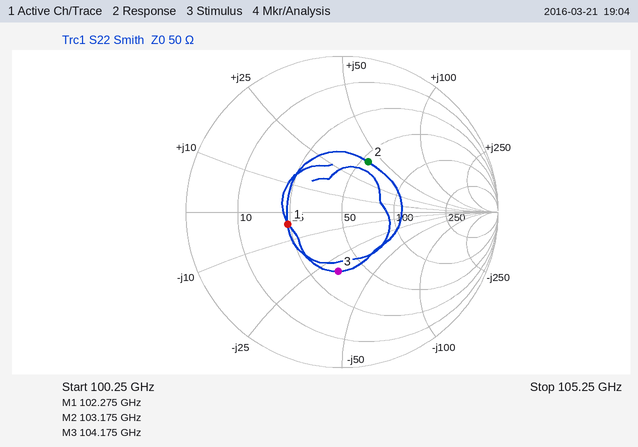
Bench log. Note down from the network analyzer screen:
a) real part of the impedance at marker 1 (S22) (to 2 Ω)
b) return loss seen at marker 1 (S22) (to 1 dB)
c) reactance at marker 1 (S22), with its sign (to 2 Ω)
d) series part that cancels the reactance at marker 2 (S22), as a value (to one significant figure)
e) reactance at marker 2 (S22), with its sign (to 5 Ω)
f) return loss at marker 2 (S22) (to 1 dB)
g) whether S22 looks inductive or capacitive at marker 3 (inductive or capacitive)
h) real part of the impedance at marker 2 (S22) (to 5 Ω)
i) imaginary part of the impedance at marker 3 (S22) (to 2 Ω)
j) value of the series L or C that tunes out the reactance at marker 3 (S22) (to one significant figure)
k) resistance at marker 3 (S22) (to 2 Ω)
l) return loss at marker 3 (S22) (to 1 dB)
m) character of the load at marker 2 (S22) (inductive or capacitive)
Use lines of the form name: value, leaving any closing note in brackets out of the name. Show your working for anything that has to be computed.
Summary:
real part of the impedance at marker 1 (S22): 24 Ω
return loss seen at marker 1 (S22): 9 dB
reactance at marker 1 (S22), with its sign: -4 Ω
series part that cancels the reactance at marker 2 (S22), as a value: C = 1/(2π × 103.175 GHz × 40 Ω) ≈ 38.6 fF, so 40 fF to one significant figure
reactance at marker 2 (S22), with its sign: +40 Ω
return loss at marker 2 (S22): 9 dB
whether S22 looks inductive or capacitive at marker 3: capacitive
real part of the impedance at marker 2 (S22): 55 Ω
imaginary part of the impedance at marker 3 (S22): -32 Ω
value of the series L or C that tunes out the reactance at marker 3 (S22): L = 32 Ω/(2π × 104.175 GHz) ≈ 48.9 pH, so 50 pH to one significant figure
resistance at marker 3 (S22): 36 Ω
return loss at marker 3 (S22): 8 dB
character of the load at marker 2 (S22): inductive
